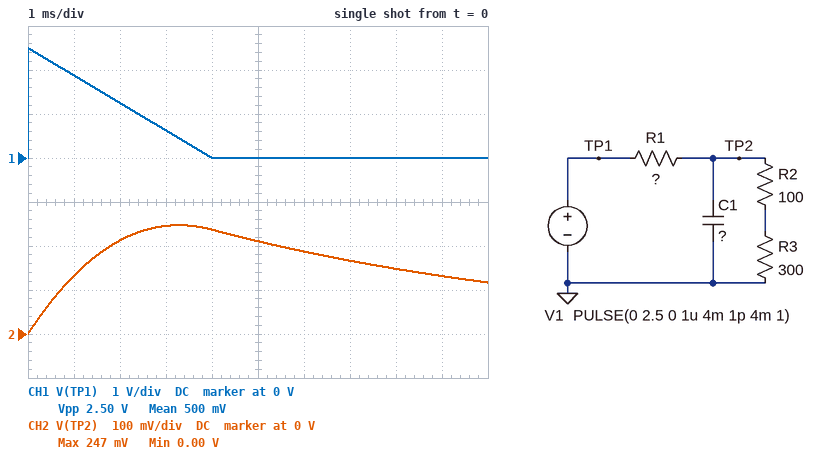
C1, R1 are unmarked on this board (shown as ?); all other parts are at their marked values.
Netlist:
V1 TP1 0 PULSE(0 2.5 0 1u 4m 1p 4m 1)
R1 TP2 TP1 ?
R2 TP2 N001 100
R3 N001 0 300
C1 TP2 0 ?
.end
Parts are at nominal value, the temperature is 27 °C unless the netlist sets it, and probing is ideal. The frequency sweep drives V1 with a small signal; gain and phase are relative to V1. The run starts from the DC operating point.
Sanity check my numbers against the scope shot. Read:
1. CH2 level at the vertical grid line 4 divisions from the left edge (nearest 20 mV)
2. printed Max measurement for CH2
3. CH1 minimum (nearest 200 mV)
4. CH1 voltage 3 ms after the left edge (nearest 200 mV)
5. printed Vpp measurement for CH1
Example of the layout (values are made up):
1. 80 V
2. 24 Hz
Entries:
1. 240 mV
2. 247 mV
3. 0 V
4. 600 mV
5. 2.50 V
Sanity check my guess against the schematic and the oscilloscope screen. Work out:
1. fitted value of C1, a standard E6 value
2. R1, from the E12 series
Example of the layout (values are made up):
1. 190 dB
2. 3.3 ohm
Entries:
1. 47 µF
2. 330 Ω
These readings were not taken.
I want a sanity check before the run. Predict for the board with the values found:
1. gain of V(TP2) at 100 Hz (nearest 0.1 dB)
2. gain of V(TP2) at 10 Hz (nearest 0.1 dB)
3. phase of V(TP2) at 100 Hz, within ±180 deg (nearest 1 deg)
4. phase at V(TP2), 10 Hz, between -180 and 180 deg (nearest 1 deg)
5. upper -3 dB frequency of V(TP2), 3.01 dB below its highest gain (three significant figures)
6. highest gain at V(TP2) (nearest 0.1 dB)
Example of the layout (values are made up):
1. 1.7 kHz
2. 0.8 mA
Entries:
1. -19.9 dB
2. -6.3 dB
3. -79 deg
4. -28 deg
5. 18.7 Hz
6. -5.2 dB
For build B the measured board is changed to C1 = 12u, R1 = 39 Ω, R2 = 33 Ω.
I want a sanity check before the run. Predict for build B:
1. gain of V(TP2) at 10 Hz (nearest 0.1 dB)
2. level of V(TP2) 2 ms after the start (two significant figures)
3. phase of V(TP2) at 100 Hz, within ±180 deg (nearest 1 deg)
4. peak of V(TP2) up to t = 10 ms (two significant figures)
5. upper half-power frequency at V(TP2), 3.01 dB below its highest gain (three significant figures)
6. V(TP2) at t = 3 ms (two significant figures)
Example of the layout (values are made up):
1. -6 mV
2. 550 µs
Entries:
1. -1.0 dB
2. 1.3 V
3. -15 deg
4. 1.7 V
5. 380 Hz
6. 790 mV
